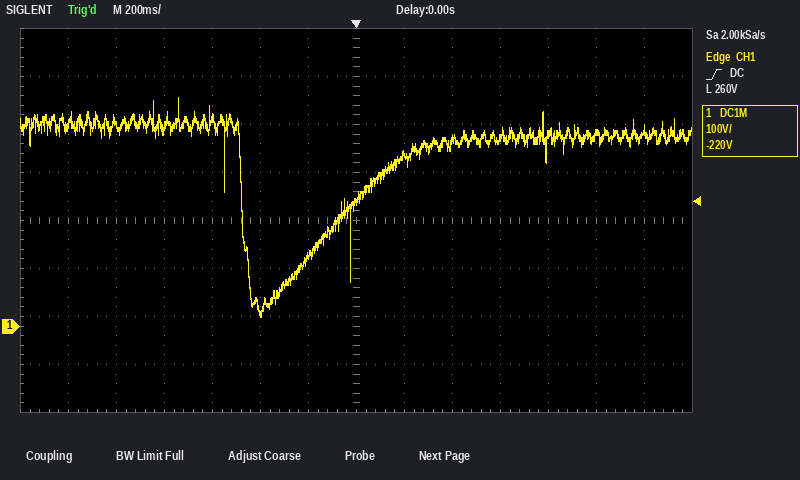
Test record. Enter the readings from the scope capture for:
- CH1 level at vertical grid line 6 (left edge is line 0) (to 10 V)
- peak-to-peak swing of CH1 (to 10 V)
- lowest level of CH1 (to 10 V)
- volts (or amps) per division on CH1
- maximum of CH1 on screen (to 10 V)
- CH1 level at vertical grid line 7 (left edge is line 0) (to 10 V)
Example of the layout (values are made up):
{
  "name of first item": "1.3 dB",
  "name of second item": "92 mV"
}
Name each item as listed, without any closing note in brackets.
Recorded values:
{
  "CH1 level at vertical grid line 6 (left edge is line 0)": "150 V",
  "peak-to-peak swing of CH1": "460 V",
  "lowest level of CH1": "20 V",
  "volts (or amps) per division on CH1": "100 V",
  "maximum of CH1 on screen": "480 V",
  "CH1 level at vertical grid line 7 (left edge is line 0)": "260 V"
}
